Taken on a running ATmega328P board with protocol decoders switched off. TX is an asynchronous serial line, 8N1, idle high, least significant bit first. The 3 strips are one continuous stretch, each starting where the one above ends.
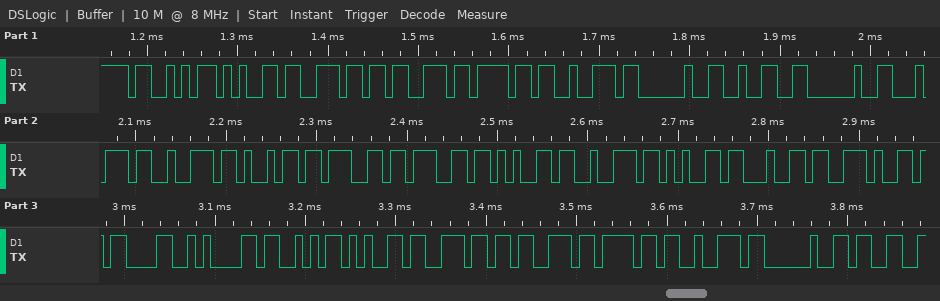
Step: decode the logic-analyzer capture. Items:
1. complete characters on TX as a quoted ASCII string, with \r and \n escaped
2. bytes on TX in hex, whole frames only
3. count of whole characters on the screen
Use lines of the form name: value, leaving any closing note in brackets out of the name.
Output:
complete characters on TX as a quoted ASCII string, with \r and \n escaped: "Sensor 2 triggered.\r\nSensor 3"
bytes on TX in hex, whole frames only: 53 65 6E 73 6F 72 20 32 20 74 72 69 67 67 65 72 65 64 2E 0D 0A 53 65 6E 73 6F 72 20 33
count of whole characters on the screen: 29
